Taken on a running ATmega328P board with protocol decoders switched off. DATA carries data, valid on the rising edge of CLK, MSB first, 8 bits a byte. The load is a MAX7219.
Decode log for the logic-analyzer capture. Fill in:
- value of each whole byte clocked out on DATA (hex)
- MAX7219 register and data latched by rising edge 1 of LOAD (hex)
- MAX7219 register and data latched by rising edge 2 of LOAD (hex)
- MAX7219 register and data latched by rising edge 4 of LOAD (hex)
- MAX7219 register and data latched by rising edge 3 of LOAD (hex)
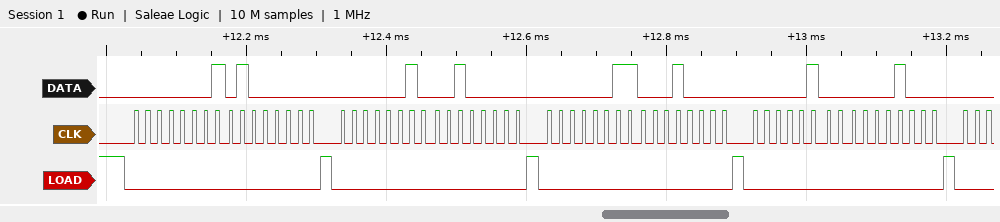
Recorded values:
01 40 02 20 03 10 04 08
register 0x1, data 0x40
register 0x2, data 0x20
register 0x4, data 0x08
register 0x3, data 0x10
